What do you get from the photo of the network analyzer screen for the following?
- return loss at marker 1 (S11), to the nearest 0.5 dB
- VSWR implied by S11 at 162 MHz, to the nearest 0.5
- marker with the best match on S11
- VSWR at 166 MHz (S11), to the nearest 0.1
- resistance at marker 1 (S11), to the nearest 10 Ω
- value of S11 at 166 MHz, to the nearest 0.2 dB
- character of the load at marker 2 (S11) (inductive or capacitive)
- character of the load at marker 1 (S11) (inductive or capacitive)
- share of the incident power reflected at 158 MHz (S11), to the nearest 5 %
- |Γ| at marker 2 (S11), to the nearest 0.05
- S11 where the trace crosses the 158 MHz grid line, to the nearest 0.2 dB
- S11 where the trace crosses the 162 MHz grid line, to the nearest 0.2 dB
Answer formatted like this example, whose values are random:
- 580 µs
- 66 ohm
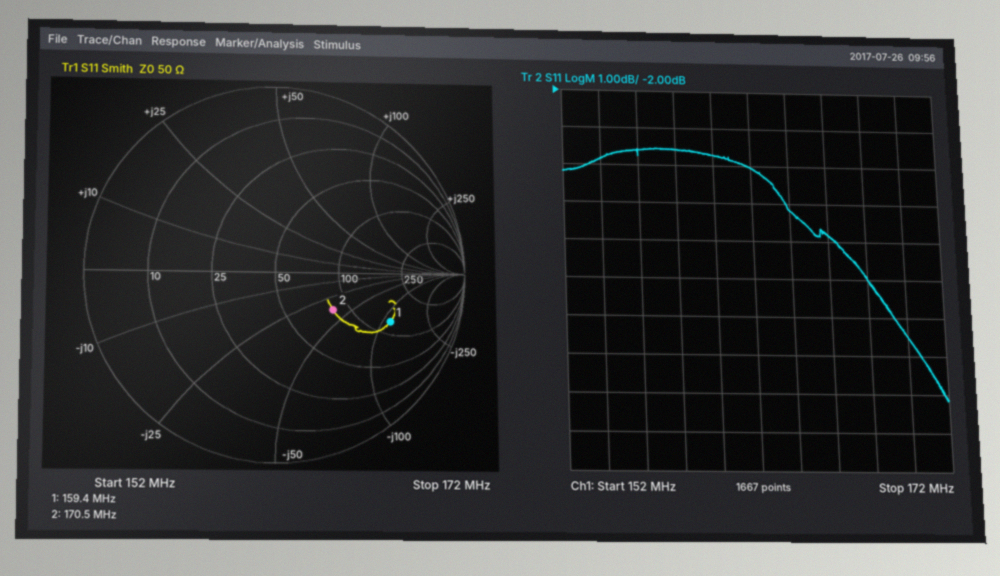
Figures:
- 3.5 dB
- 4.5
- marker 2
- 3.1
- 130 Ω
- -5.8 dB
- capacitive
- capacitive
- 45 %
- 0.35
- -3.6 dB
- -4.0 dB
